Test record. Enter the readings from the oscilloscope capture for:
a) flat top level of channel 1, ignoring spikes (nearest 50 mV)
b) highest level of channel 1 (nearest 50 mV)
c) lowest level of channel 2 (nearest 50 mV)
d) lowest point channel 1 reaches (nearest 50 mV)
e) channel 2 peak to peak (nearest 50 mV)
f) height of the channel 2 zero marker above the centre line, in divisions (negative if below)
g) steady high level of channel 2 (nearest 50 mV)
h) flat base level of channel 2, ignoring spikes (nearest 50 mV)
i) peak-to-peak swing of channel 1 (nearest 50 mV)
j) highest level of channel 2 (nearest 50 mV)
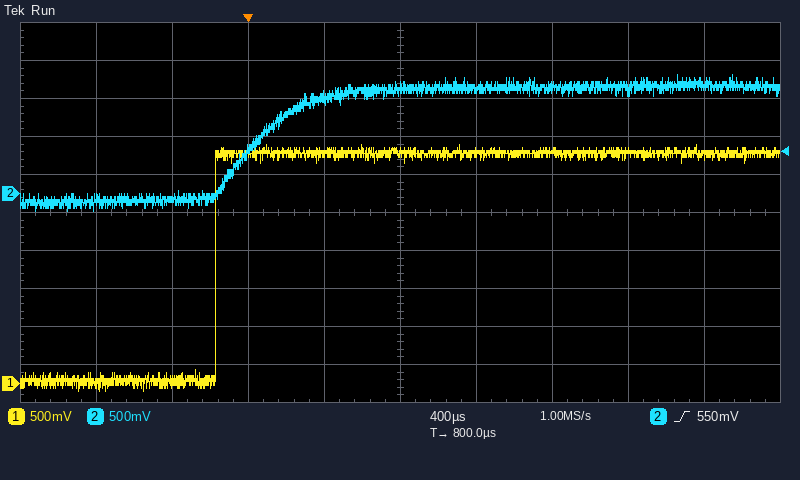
3.00 V
3.15 V
-250 mV
-100 mV
1.80 V
+0.5 div
1.40 V
-100 mV
3.25 V
1.55 V
